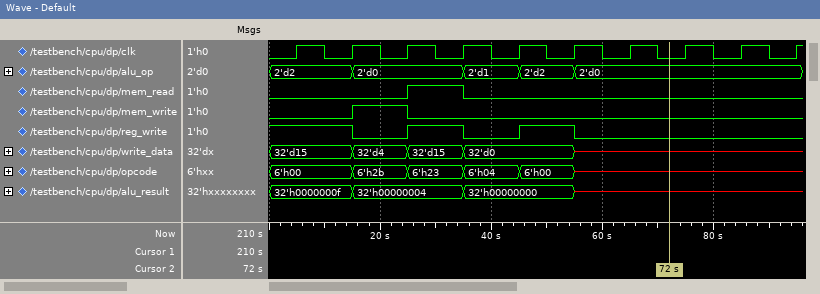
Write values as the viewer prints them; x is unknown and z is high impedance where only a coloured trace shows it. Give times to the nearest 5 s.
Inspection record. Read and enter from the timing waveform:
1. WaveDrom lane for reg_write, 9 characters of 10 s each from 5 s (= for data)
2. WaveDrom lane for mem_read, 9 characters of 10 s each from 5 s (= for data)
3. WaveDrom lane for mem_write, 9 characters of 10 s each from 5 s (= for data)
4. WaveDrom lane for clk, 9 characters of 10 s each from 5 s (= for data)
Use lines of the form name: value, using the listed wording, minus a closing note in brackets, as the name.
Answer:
WaveDrom lane for reg_write, 9 characters of 10 s each from 5 s: {name: 'reg_write', wave: '101010...'}
WaveDrom lane for mem_read, 9 characters of 10 s each from 5 s: {name: 'mem_read', wave: '0.10.....'}
WaveDrom lane for mem_write, 9 characters of 10 s each from 5 s: {name: 'mem_write', wave: '010......'}
WaveDrom lane for clk, 9 characters of 10 s each from 5 s: {name: 'clk', wave: 'p........'}
